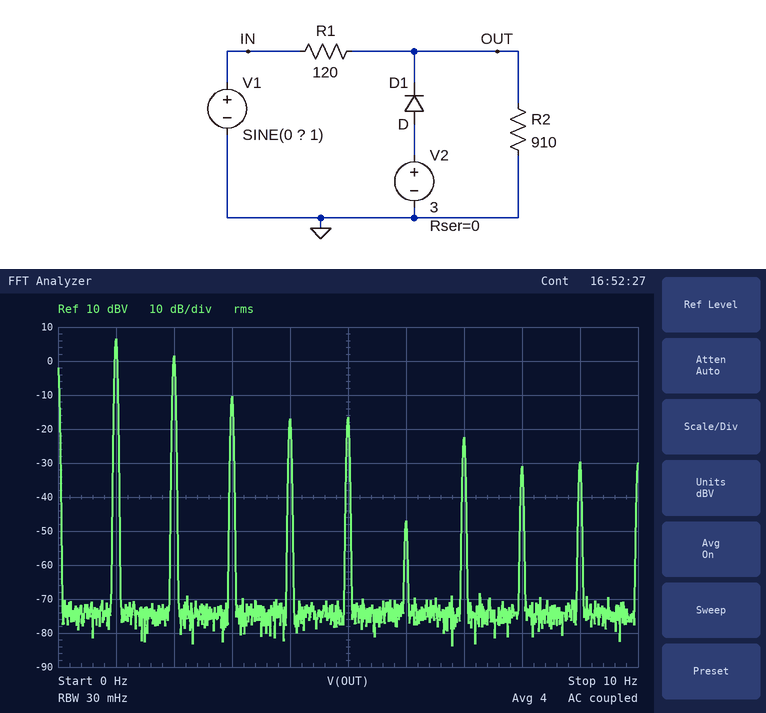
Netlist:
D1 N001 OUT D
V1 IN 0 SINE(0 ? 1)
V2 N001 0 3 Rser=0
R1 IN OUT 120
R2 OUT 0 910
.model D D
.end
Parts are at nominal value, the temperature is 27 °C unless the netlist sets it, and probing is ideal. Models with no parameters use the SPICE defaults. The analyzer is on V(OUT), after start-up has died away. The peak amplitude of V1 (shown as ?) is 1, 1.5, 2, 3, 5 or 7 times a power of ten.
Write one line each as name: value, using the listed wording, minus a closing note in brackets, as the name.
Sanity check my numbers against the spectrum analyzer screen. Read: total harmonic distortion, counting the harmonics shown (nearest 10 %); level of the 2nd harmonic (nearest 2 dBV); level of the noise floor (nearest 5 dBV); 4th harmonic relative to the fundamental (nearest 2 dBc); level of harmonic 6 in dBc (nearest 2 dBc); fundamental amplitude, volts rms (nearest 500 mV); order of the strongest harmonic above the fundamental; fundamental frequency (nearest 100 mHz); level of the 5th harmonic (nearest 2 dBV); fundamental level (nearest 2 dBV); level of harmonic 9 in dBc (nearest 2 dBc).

total harmonic distortion, counting the harmonics shown: 60 %
level of the 2nd harmonic: 2 dBV
level of the noise floor: -75 dBV
4th harmonic relative to the fundamental: -24 dBc
level of harmonic 6 in dBc: -54 dBc
fundamental amplitude, volts rms: 2.0 V
order of the strongest harmonic above the fundamental: 2
fundamental frequency: 1.0 Hz
level of the 5th harmonic: -16 dBV
fundamental level: 6 dBV
level of harmonic 9 in dBc: -36 dBc
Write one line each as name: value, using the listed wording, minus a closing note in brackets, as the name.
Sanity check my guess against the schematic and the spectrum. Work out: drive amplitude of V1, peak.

drive amplitude of V1, peak: 10 V
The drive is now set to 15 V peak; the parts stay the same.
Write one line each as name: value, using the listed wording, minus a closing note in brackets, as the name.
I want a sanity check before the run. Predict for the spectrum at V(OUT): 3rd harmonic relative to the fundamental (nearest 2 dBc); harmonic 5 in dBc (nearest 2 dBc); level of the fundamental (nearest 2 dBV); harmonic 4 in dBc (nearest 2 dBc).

3rd harmonic relative to the fundamental: -22 dBc
harmonic 5 in dBc: -26 dBc
level of the fundamental: 12 dBV
harmonic 4 in dBc: -22 dBc
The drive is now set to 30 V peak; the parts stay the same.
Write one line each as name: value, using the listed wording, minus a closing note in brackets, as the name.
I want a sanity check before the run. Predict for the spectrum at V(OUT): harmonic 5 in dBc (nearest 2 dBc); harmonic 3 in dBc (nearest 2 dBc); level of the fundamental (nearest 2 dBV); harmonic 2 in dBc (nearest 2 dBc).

harmonic 5 in dBc: -32 dBc
harmonic 3 in dBc: -28 dBc
level of the fundamental: 18 dBV
harmonic 2 in dBc: -6 dBc
